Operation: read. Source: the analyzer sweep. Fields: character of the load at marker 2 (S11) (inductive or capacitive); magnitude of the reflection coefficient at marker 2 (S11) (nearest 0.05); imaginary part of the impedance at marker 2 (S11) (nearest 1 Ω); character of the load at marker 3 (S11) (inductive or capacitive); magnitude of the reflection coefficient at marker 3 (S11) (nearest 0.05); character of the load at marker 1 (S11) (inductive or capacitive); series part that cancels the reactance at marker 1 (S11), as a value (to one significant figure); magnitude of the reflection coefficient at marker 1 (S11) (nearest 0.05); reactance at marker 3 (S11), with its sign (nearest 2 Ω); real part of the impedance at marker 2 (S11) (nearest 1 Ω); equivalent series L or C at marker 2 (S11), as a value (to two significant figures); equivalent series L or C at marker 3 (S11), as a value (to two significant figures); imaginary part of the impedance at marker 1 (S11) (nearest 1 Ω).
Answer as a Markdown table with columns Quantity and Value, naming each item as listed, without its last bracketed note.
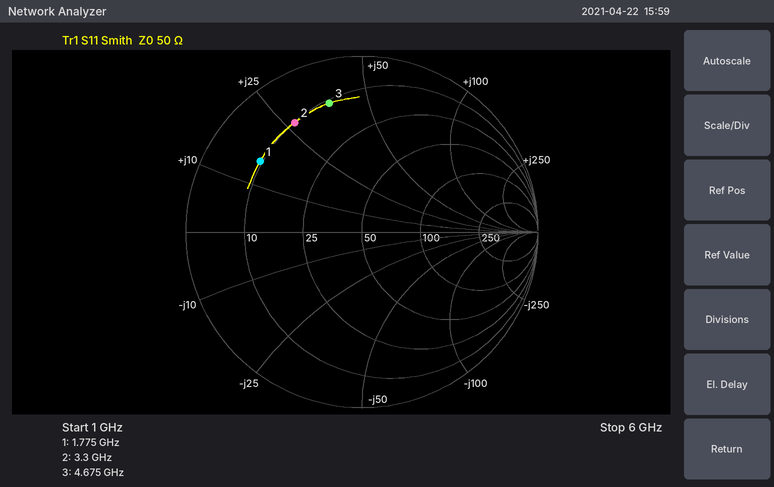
| Quantity | Value |
|---|---|
| character of the load at marker 2 (S11) | inductive |
| magnitude of the reflection coefficient at marker 2 (S11) | 0.75 |
| imaginary part of the impedance at marker 2 (S11) | +27 Ω |
| character of the load at marker 3 (S11) | inductive |
| magnitude of the reflection coefficient at marker 3 (S11) | 0.75 |
| character of the load at marker 1 (S11) | inductive |
| series part that cancels the reactance at marker 1 (S11), as a value | 6 pF |
| magnitude of the reflection coefficient at marker 1 (S11) | 0.70 |
| reactance at marker 3 (S11), with its sign | +38 Ω |
| real part of the impedance at marker 2 (S11) | 10 Ω |
| equivalent series L or C at marker 2 (S11), as a value | 1.3 nH |
| equivalent series L or C at marker 3 (S11), as a value | 1.3 nH |
| imaginary part of the impedance at marker 1 (S11) | +15 Ω |
